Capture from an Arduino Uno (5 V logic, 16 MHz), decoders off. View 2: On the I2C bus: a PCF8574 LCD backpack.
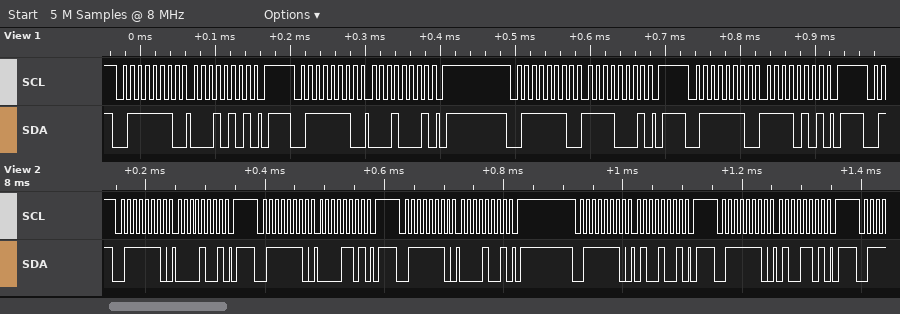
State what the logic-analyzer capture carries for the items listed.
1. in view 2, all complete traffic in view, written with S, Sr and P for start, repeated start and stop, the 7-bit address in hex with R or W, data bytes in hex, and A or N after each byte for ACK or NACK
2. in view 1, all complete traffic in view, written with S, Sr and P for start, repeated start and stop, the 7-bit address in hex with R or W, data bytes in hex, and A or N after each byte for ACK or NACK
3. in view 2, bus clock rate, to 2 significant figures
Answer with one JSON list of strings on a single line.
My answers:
["S 3FW A 09 A P S 3FW A 0D A P S 3FW A 09 A P S 3FW A 49 A P S 3FW A 4D A P", "S 3FW A 15 A P S 3FW A 11 A P S 3FW A F1 A P S 3FW A F5 A P", "100 kHz"]
